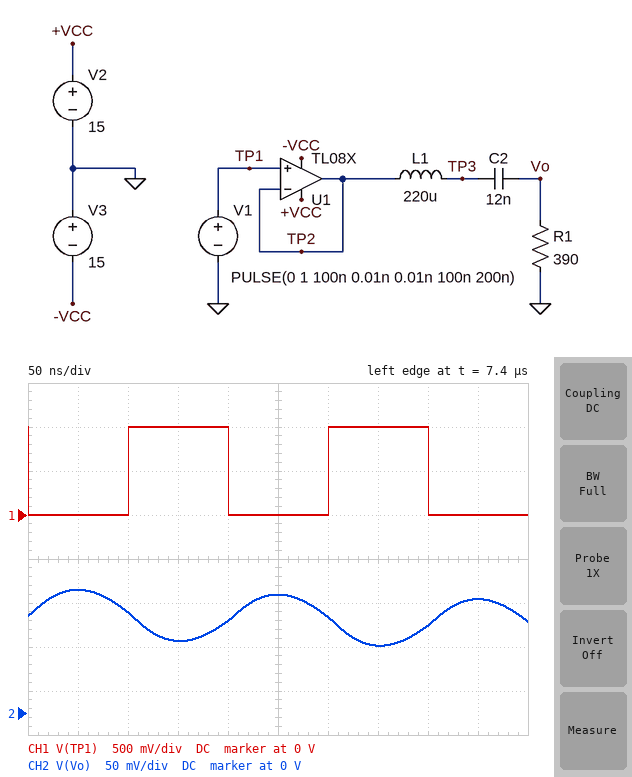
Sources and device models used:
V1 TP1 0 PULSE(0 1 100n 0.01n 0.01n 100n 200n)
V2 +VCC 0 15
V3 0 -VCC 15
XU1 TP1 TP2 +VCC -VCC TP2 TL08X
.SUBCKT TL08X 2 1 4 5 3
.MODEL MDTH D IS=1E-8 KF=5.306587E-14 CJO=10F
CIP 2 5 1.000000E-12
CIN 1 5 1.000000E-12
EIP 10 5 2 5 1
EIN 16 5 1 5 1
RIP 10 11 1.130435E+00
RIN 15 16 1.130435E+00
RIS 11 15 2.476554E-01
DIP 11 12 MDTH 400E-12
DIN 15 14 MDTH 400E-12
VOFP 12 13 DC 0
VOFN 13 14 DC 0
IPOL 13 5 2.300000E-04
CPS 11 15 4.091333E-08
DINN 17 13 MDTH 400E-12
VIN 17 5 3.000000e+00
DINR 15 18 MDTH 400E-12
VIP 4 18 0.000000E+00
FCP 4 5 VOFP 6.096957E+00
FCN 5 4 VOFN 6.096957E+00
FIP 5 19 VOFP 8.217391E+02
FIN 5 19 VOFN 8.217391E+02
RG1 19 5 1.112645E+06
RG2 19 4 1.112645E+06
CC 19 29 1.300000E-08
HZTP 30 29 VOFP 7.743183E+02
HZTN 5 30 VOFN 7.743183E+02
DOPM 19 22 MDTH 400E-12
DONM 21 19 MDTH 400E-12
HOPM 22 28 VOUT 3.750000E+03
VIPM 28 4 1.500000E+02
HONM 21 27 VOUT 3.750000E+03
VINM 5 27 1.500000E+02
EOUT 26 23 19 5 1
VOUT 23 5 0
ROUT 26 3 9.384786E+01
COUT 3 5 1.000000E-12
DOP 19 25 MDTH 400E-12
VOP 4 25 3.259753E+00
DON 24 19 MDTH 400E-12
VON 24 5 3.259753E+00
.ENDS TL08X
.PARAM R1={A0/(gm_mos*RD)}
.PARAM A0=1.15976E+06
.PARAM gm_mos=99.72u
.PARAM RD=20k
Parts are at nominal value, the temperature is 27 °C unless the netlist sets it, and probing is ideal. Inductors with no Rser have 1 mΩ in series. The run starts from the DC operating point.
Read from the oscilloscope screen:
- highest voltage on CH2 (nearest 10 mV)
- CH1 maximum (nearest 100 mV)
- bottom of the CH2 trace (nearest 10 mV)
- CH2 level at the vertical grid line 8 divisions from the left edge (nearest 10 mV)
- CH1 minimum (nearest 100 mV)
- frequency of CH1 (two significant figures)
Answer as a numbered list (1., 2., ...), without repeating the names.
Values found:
1. 140 mV
2. 1.0 V
3. 80 mV
4. 100 mV
5. 0 V
6. 5.0 MHz
